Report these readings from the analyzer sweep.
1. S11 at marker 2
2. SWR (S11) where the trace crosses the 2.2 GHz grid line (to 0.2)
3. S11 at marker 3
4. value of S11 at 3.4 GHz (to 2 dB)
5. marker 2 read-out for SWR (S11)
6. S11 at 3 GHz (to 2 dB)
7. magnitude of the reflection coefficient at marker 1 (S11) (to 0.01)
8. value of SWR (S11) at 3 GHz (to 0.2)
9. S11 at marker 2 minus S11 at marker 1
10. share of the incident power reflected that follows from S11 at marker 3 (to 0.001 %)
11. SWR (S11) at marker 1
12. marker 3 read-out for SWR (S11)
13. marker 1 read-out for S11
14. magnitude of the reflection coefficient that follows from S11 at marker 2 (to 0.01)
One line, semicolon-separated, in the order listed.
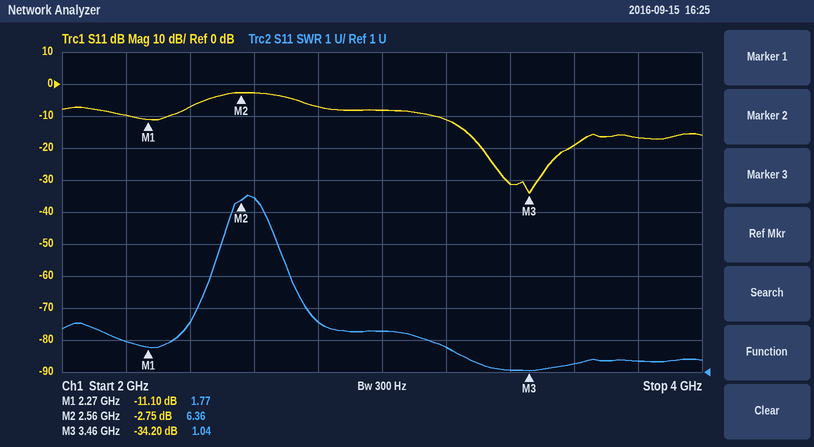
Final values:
-2.75 dB; 2.0; -34.20 dB; -32 dB; 6.36; -8 dB; 0.28; 2.2; 8.35 dB; 0.038 %; 1.77; 1.04; -11.10 dB; 0.73
